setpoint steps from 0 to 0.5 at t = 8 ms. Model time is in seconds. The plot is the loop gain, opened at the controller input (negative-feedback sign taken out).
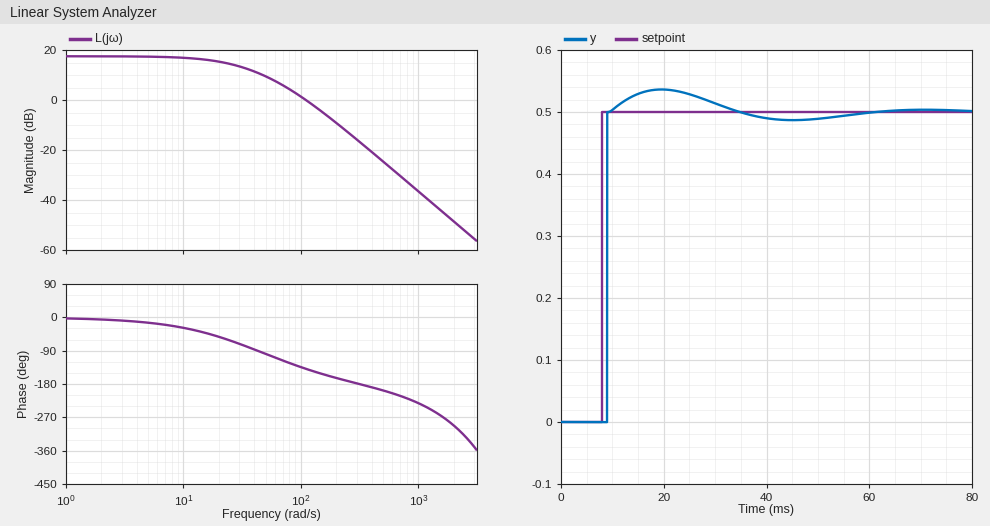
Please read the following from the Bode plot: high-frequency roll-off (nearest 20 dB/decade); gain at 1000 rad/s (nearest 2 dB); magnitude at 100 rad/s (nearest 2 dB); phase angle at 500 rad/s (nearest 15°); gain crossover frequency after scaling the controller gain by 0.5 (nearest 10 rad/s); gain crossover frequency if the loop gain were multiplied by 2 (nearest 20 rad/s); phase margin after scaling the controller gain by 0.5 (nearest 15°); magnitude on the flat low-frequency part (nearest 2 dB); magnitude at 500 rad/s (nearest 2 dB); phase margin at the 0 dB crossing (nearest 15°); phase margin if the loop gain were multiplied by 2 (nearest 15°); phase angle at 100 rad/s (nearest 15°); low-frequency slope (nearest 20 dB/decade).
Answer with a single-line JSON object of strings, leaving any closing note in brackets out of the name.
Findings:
{"high-frequency roll-off": "-40 dB/decade", "gain at 1000 rad/s": "-36 dB", "magnitude at 100 rad/s": "2 dB", "phase angle at 500 rad/s": "-195°", "gain crossover frequency after scaling the controller gain by 0.5": "70 rad/s", "gain crossover frequency if the loop gain were multiplied by 2": "160 rad/s", "phase margin after scaling the controller gain by 0.5": "60°", "magnitude on the flat low-frequency part": "18 dB", "magnitude at 500 rad/s": "-24 dB", "phase margin at the 0 dB crossing": "45°", "phase margin if the loop gain were multiplied by 2": "30°", "phase angle at 100 rad/s": "-135°", "low-frequency slope": "0 dB/decade"}
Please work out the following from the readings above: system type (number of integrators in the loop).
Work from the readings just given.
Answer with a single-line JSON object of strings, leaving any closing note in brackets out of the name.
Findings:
{"system type": "0"}
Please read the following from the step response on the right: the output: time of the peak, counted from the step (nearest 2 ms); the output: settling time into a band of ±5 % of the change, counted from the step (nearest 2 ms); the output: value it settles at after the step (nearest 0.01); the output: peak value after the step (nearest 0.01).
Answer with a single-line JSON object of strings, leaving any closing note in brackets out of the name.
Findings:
{"the output: time of the peak, counted from the step": "12 ms", "the output: settling time into a band of ±5 % of the change, counted from the step": "18 ms", "the output: value it settles at after the step": "0.50", "the output: peak value after the step": "0.54"}
